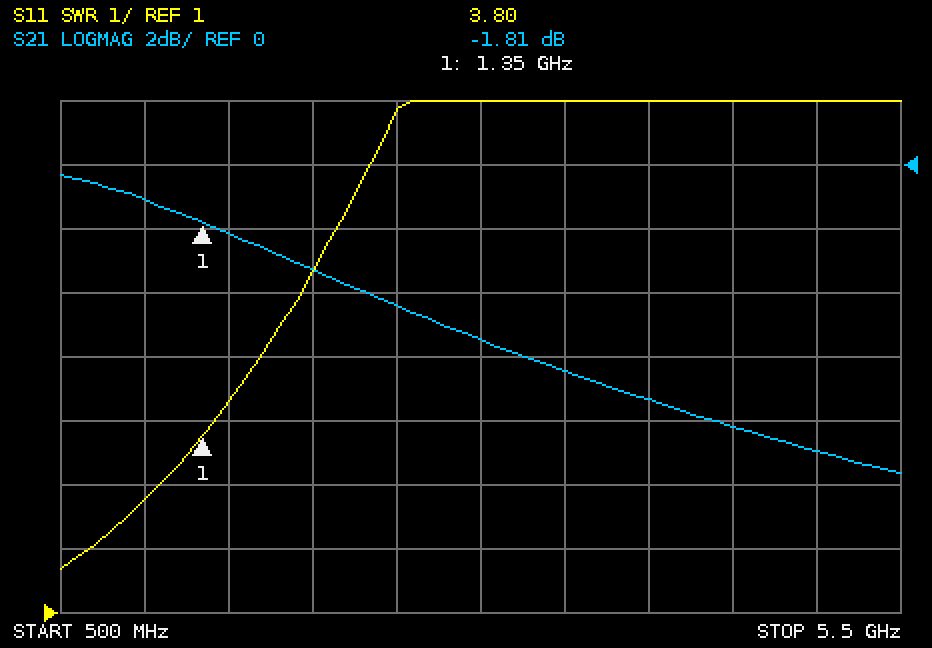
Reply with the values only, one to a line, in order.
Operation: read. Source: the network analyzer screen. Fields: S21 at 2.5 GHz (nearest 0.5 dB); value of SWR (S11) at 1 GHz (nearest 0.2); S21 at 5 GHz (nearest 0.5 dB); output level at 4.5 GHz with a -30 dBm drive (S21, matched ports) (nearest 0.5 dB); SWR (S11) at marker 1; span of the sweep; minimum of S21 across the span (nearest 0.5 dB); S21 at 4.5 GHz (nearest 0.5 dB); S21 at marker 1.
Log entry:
-4.5 dB
2.8
-9.0 dB
-38.0 dBm
3.80
5 GHz
-9.5 dB
-8.0 dB
-1.81 dB
